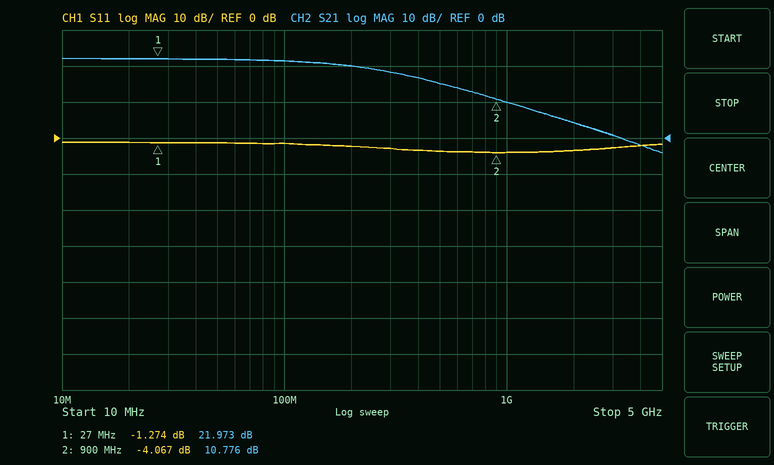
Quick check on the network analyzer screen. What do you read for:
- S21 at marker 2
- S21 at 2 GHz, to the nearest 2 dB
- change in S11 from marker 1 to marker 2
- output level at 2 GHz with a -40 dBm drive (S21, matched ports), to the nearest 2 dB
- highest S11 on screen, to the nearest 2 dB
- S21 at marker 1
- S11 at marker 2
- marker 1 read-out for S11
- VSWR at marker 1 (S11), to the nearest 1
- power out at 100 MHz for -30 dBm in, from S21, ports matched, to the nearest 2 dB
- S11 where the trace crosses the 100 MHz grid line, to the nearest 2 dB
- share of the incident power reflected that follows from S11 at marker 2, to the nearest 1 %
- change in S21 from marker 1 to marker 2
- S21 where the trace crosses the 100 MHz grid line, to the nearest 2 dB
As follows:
10.776 dB
4 dB
-2.793 dB
-36 dBm
-2 dB
21.973 dB
-4.067 dB
-1.274 dB
14
-8 dBm
-2 dB
39 %
-11.197 dB
22 dB
